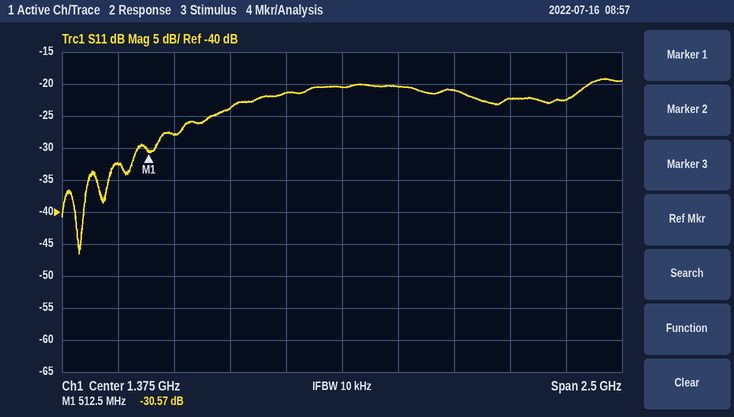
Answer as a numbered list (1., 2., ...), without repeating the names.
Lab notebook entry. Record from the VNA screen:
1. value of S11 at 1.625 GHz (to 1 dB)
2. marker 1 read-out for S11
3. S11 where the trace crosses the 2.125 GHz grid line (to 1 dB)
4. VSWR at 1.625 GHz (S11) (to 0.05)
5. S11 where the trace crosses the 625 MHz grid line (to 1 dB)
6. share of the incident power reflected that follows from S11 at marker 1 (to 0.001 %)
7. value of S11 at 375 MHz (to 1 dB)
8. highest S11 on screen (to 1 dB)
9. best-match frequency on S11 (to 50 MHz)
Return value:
1. -20 dB
2. -30.57 dB
3. -22 dB
4. 1.20
5. -28 dB
6. 0.088 %
7. -32 dB
8. -19 dB
9. 200 MHz
